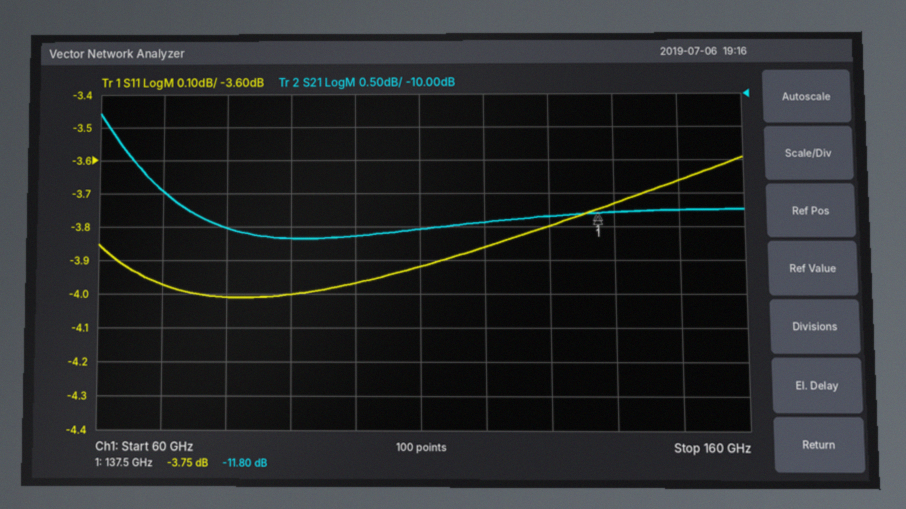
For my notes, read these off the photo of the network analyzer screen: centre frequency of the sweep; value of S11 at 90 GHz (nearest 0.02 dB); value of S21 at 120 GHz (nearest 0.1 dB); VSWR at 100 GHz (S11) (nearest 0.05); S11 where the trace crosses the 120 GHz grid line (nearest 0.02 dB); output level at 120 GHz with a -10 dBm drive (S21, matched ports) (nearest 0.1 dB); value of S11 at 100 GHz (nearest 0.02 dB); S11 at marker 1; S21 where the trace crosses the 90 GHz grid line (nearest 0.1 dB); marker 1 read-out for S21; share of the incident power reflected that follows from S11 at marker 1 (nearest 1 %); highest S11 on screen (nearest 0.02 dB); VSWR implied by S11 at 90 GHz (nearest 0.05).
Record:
110 GHz
-4.00 dB
-11.9 dB
4.45
-3.86 dB
-21.9 dBm
-3.96 dB
-3.75 dB
-12.2 dB
-11.80 dB
42 %
-3.60 dB
4.40
